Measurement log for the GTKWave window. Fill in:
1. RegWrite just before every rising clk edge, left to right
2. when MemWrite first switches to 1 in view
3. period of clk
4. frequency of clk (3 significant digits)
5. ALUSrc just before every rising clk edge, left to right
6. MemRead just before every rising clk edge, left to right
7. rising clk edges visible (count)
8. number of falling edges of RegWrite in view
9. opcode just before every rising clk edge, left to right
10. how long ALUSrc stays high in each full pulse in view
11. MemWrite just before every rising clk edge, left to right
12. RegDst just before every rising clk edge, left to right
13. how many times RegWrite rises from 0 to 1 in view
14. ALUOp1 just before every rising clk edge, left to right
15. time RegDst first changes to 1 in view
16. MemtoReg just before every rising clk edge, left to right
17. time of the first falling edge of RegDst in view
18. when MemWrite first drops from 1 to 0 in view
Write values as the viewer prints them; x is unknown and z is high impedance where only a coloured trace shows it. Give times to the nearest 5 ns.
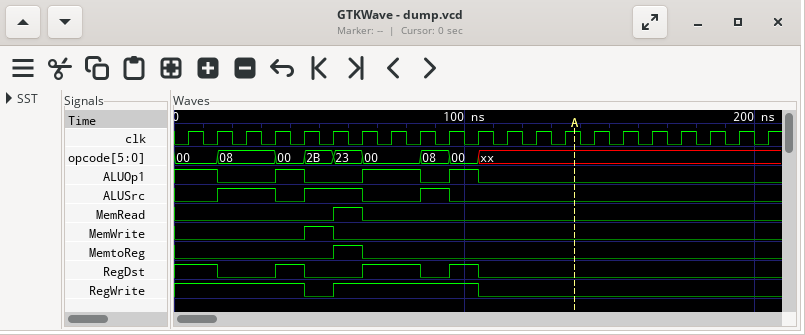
1 1 1 1 1 0 1 1 1 1 1 0 0 0 0 0 0 0 0 0 0
45 ns
10 ns
100 MHz
0 0 1 1 0 1 1 0 0 1 0 0 0 0 0 0 0 0 0 0 0
0 0 0 0 0 0 1 0 0 0 0 0 0 0 0 0 0 0 0 0 0
21
2
00, 00, 08, 08, 00, 2B, 23, 00, 00, 08, 00, xx, xx, xx, xx, xx, xx, xx, xx, xx, xx
20 ns, 20 ns, 10 ns
0 0 0 0 0 1 0 0 0 0 0 0 0 0 0 0 0 0 0 0 0
1 1 0 0 1 0 0 1 1 0 1 0 0 0 0 0 0 0 0 0 0
1
1 1 0 0 1 0 0 1 1 0 1 0 0 0 0 0 0 0 0 0 0
35 ns
0 0 0 0 0 0 1 0 0 0 0 0 0 0 0 0 0 0 0 0 0
15 ns
55 ns
